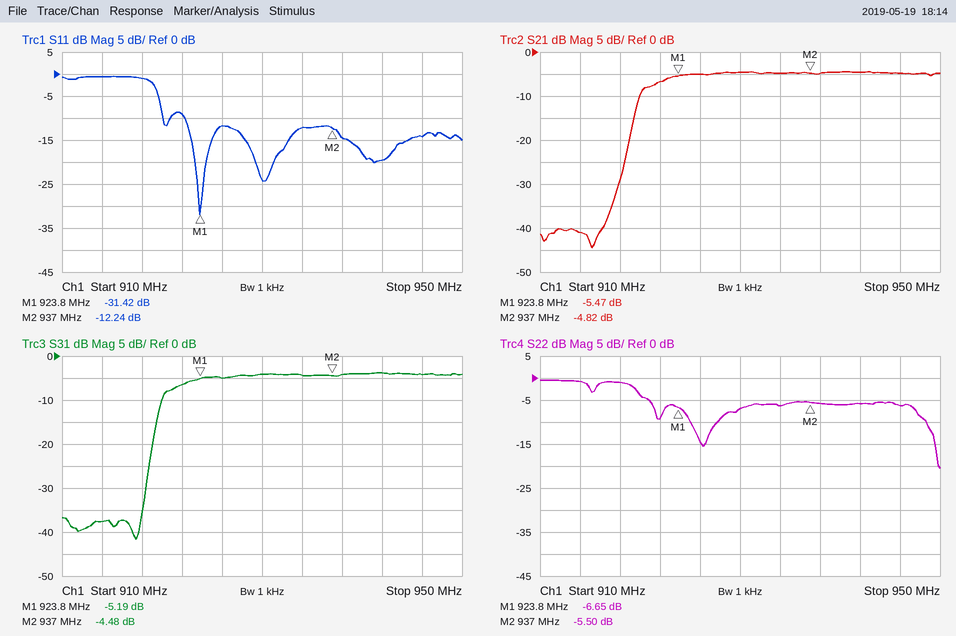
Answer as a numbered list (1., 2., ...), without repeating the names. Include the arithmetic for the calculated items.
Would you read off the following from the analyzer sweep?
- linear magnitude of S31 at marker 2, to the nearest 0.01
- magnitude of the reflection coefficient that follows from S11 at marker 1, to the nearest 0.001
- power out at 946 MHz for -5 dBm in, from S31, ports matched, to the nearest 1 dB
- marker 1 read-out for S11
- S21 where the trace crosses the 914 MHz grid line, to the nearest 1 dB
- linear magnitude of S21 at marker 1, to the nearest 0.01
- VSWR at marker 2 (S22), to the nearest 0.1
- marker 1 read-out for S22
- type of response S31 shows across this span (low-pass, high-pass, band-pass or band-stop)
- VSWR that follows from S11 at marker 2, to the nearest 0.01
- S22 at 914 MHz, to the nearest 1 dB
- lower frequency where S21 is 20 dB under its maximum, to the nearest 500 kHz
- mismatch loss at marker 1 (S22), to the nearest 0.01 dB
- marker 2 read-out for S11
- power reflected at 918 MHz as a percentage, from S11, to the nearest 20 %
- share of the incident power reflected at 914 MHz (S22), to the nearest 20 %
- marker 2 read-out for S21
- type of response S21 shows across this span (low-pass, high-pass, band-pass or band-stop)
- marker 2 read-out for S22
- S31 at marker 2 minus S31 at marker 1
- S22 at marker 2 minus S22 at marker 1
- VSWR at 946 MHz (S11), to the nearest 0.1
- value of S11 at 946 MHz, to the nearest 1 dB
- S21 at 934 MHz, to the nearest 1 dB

1. 10^(-4.48/20) ≈ 0.60
2. 10^(-31.42/20) ≈ 0.027
3. -5 dBm + (-4 dB) = -9 dBm
4. -31.42 dB
5. -41 dB
6. 10^(-5.47/20) ≈ 0.53
7. (1 + 0.5309)/(1 − 0.5309) ≈ 3.3
8. -6.65 dB
9. high-pass
10. (1 + 0.2443)/(1 − 0.2443) ≈ 1.65
11. -1 dB
12. 918.5 MHz
13. −10 log10(1 − 10^(-6.65/10)) ≈ 1.06 dB
14. -12.24 dB
15. 10^(-1/10) ≈ 79.4 %, so 80 % to the nearest 20 %
16. 10^(-1/10) ≈ 79.4 %, so 80 % to the nearest 20 %
17. -4.82 dB
18. high-pass
19. -5.50 dB
20. -4.48 − (-5.19) = 0.71 dB
21. -5.5 − (-6.65) = 1.15 dB
22. |Γ| = 10^(-14/20) = 0.1995; VSWR = (1 + 0.1995)/(1 − 0.1995) ≈ 1.5
23. -14 dB
24. -5 dB
